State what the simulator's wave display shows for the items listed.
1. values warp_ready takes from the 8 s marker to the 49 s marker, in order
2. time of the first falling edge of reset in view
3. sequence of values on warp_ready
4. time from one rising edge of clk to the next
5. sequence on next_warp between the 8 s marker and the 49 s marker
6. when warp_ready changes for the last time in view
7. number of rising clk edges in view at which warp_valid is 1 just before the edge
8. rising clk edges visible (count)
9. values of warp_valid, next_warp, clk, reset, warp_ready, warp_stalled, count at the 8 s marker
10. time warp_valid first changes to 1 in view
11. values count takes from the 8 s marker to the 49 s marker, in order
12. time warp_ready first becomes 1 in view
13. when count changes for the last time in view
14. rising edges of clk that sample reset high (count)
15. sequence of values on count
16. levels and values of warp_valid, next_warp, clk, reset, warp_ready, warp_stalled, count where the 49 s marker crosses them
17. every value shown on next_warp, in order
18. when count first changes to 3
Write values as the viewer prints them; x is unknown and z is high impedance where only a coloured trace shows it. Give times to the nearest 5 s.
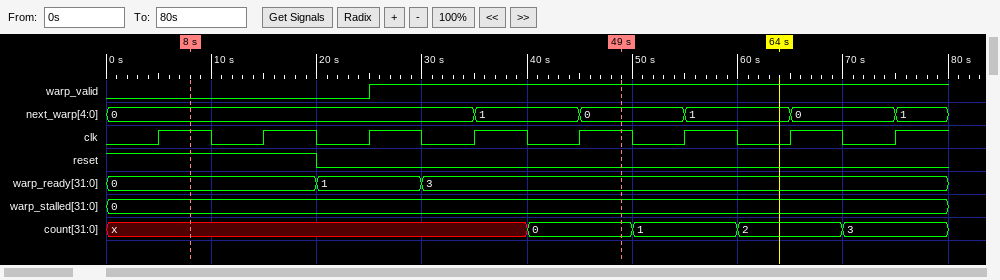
0, 1, 3
20 s
0, 1, 3
10 s
0, 1, 0
30 s
5
8
warp_valid=0, next_warp=0, clk=1, reset=1, warp_ready=0, warp_stalled=0, count=x
25 s
x, 0
20 s
70 s
2
x, 0, 1, 2, 3
warp_valid=1, next_warp=0, clk=1, reset=0, warp_ready=3, warp_stalled=0, count=0
0, 1, 0, 1, 0, 1
70 s
